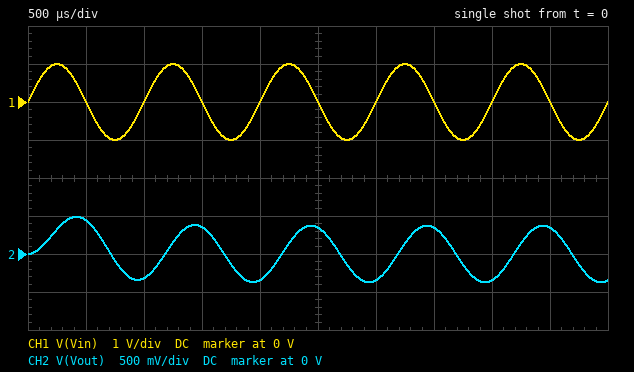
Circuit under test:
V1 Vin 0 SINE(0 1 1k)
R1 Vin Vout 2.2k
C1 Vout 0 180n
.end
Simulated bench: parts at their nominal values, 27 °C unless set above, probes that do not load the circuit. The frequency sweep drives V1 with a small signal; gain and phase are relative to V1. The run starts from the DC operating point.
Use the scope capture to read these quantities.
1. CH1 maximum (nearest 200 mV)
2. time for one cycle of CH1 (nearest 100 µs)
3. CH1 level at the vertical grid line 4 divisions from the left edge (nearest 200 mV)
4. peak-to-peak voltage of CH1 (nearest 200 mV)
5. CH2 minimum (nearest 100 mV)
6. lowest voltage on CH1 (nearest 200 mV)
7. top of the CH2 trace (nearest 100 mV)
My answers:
1.0 V
1.0 ms
0 V
2.0 V
-400 mV
-1.0 V
500 mV
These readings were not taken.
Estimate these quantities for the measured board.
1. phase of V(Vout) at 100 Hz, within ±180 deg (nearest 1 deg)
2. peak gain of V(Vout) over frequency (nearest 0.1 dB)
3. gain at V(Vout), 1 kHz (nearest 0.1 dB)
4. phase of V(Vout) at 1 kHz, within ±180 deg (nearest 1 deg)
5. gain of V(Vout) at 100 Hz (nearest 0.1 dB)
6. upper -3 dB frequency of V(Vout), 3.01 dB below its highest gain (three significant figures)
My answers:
-14 deg
0 dB
-8.6 dB
-68 deg
-0.3 dB
402 Hz
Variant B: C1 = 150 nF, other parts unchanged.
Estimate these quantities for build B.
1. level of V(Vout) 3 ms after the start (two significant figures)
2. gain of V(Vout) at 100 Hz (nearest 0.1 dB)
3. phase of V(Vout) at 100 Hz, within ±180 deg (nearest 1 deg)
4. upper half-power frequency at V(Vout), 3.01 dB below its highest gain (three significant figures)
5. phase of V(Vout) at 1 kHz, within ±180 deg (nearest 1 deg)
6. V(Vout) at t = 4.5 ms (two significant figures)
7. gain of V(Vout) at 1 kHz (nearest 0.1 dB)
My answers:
-390 mV
-0.2 dB
-12 deg
482 Hz
-64 deg
390 mV
-7.2 dB
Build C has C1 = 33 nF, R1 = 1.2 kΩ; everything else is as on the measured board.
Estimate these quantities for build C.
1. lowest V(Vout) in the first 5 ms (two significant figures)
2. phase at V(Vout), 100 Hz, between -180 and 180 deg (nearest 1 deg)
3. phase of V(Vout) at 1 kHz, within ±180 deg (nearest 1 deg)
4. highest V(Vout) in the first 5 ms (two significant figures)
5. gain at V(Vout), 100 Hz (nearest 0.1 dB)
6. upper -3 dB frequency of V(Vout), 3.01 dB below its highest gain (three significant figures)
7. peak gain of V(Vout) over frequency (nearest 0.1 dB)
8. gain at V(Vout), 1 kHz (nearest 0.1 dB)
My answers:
-970 mV
-1 deg
-14 deg
970 mV
0 dB
4.02 kHz
0 dB
-0.3 dB
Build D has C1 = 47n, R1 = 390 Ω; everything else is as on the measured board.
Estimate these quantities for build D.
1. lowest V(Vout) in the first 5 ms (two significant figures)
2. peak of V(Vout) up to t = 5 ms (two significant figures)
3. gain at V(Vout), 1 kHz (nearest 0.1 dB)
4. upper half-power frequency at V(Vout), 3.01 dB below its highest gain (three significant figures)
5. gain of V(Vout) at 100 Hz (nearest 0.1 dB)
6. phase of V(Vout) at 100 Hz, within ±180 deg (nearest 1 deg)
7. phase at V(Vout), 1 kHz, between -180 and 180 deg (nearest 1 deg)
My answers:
-990 mV
990 mV
-0.1 dB
8.68 kHz
0 dB
-1 deg
-7 deg
